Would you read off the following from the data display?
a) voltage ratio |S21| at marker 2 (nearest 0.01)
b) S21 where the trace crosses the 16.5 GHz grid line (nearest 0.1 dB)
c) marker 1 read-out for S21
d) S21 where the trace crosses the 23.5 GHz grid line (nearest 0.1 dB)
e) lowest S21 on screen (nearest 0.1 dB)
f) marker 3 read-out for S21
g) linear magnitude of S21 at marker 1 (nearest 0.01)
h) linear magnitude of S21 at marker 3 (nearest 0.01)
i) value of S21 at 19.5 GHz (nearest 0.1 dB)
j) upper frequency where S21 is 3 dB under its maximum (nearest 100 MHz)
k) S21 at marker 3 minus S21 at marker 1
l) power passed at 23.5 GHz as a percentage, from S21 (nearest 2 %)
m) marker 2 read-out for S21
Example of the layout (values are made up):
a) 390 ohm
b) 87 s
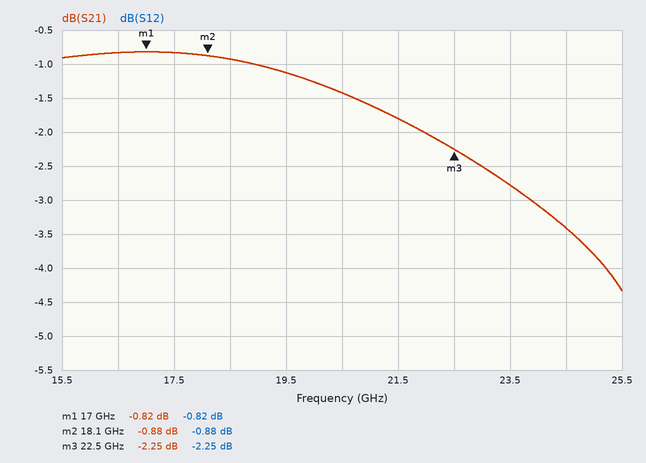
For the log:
a) 0.90
b) -0.8 dB
c) -0.82 dB
d) -2.8 dB
e) -4.3 dB
f) -2.25 dB
g) 0.91
h) 0.77
i) -1.1 dB
j) 25.0 GHz
k) -1.43 dB
l) 52 %
m) -0.88 dB
